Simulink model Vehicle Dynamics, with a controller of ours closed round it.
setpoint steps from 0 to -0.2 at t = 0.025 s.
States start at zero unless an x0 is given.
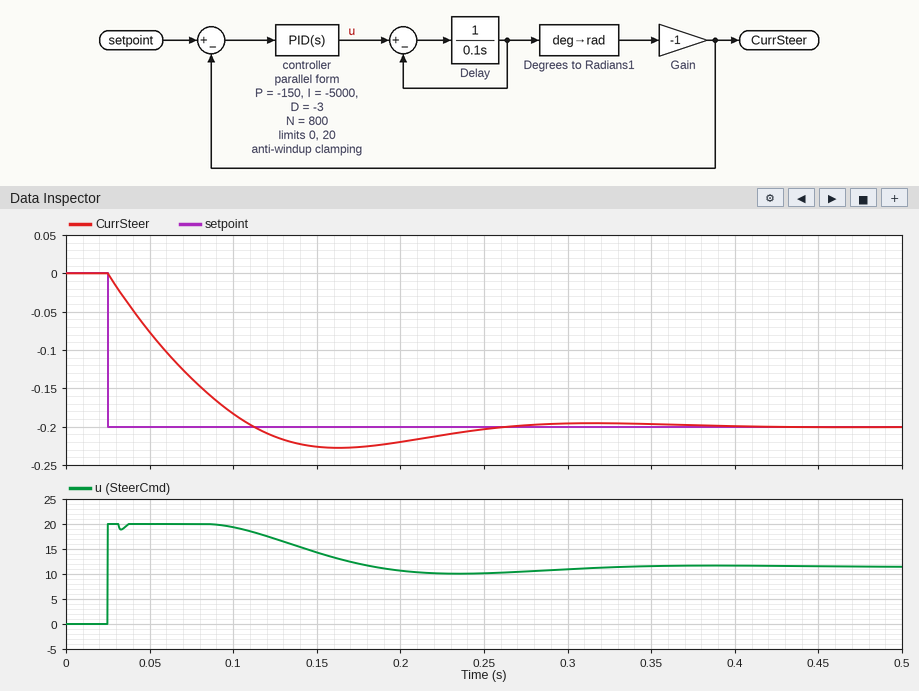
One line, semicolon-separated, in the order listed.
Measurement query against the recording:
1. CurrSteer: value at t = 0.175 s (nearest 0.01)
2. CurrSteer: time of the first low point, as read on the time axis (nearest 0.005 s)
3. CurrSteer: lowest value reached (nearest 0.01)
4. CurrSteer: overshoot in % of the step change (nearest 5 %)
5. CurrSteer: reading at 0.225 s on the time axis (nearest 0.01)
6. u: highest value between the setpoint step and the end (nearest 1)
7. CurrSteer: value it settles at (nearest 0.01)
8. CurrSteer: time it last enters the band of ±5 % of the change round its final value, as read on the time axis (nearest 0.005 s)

-0.23; 0.165 s; -0.23; 15 %; -0.21; 20; -0.20; 0.230 s
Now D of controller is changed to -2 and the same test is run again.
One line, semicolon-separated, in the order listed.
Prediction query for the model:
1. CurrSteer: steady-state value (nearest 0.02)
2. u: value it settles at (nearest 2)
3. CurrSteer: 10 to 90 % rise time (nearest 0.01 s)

-0.20; 12; 0.07 s
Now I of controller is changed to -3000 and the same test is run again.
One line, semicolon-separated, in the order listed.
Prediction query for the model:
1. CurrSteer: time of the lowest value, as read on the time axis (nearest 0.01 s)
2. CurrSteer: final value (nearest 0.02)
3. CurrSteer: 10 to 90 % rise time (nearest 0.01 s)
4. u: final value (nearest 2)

0.18 s; -0.20; 0.07 s; 12
